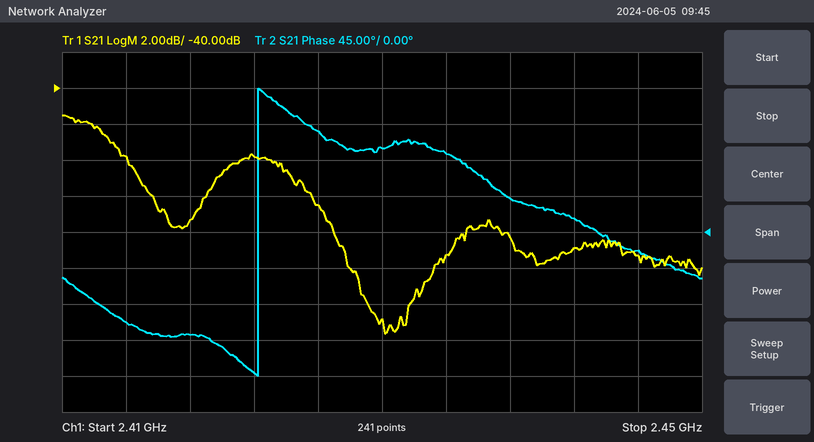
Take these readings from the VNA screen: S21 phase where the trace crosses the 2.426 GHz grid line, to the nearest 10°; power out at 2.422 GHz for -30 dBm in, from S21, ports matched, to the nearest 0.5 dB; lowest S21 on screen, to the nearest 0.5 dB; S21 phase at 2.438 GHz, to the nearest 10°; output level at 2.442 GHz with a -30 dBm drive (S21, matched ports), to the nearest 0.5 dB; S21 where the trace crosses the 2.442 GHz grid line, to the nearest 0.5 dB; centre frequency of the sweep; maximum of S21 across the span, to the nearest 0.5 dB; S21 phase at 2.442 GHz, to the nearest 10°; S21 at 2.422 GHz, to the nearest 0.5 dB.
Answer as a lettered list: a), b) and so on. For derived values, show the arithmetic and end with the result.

a) 130°
b) -30 dBm + (-44.0 dB) = -74.0 dBm
c) -53.5 dB
d) 40°
e) -30 dBm + (-49.0 dB) = -79.0 dBm
f) -49.0 dB
g) 2.43 GHz
h) -41.5 dB
i) 20°
j) -44.0 dB
